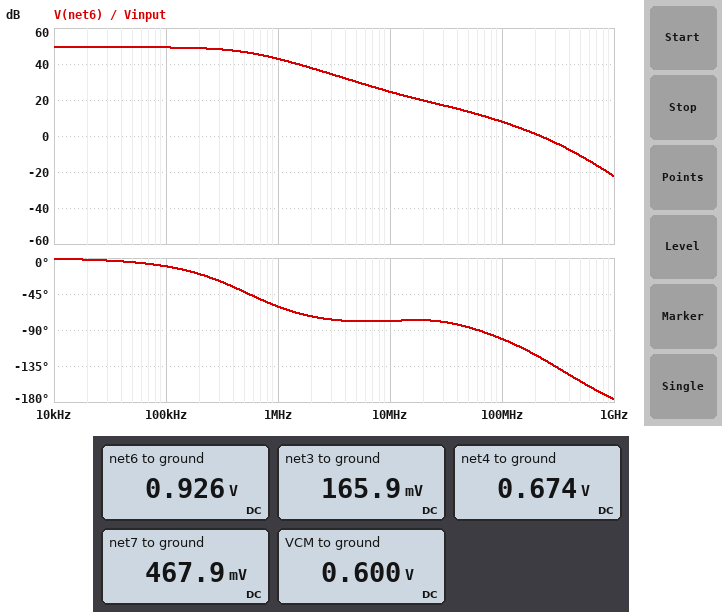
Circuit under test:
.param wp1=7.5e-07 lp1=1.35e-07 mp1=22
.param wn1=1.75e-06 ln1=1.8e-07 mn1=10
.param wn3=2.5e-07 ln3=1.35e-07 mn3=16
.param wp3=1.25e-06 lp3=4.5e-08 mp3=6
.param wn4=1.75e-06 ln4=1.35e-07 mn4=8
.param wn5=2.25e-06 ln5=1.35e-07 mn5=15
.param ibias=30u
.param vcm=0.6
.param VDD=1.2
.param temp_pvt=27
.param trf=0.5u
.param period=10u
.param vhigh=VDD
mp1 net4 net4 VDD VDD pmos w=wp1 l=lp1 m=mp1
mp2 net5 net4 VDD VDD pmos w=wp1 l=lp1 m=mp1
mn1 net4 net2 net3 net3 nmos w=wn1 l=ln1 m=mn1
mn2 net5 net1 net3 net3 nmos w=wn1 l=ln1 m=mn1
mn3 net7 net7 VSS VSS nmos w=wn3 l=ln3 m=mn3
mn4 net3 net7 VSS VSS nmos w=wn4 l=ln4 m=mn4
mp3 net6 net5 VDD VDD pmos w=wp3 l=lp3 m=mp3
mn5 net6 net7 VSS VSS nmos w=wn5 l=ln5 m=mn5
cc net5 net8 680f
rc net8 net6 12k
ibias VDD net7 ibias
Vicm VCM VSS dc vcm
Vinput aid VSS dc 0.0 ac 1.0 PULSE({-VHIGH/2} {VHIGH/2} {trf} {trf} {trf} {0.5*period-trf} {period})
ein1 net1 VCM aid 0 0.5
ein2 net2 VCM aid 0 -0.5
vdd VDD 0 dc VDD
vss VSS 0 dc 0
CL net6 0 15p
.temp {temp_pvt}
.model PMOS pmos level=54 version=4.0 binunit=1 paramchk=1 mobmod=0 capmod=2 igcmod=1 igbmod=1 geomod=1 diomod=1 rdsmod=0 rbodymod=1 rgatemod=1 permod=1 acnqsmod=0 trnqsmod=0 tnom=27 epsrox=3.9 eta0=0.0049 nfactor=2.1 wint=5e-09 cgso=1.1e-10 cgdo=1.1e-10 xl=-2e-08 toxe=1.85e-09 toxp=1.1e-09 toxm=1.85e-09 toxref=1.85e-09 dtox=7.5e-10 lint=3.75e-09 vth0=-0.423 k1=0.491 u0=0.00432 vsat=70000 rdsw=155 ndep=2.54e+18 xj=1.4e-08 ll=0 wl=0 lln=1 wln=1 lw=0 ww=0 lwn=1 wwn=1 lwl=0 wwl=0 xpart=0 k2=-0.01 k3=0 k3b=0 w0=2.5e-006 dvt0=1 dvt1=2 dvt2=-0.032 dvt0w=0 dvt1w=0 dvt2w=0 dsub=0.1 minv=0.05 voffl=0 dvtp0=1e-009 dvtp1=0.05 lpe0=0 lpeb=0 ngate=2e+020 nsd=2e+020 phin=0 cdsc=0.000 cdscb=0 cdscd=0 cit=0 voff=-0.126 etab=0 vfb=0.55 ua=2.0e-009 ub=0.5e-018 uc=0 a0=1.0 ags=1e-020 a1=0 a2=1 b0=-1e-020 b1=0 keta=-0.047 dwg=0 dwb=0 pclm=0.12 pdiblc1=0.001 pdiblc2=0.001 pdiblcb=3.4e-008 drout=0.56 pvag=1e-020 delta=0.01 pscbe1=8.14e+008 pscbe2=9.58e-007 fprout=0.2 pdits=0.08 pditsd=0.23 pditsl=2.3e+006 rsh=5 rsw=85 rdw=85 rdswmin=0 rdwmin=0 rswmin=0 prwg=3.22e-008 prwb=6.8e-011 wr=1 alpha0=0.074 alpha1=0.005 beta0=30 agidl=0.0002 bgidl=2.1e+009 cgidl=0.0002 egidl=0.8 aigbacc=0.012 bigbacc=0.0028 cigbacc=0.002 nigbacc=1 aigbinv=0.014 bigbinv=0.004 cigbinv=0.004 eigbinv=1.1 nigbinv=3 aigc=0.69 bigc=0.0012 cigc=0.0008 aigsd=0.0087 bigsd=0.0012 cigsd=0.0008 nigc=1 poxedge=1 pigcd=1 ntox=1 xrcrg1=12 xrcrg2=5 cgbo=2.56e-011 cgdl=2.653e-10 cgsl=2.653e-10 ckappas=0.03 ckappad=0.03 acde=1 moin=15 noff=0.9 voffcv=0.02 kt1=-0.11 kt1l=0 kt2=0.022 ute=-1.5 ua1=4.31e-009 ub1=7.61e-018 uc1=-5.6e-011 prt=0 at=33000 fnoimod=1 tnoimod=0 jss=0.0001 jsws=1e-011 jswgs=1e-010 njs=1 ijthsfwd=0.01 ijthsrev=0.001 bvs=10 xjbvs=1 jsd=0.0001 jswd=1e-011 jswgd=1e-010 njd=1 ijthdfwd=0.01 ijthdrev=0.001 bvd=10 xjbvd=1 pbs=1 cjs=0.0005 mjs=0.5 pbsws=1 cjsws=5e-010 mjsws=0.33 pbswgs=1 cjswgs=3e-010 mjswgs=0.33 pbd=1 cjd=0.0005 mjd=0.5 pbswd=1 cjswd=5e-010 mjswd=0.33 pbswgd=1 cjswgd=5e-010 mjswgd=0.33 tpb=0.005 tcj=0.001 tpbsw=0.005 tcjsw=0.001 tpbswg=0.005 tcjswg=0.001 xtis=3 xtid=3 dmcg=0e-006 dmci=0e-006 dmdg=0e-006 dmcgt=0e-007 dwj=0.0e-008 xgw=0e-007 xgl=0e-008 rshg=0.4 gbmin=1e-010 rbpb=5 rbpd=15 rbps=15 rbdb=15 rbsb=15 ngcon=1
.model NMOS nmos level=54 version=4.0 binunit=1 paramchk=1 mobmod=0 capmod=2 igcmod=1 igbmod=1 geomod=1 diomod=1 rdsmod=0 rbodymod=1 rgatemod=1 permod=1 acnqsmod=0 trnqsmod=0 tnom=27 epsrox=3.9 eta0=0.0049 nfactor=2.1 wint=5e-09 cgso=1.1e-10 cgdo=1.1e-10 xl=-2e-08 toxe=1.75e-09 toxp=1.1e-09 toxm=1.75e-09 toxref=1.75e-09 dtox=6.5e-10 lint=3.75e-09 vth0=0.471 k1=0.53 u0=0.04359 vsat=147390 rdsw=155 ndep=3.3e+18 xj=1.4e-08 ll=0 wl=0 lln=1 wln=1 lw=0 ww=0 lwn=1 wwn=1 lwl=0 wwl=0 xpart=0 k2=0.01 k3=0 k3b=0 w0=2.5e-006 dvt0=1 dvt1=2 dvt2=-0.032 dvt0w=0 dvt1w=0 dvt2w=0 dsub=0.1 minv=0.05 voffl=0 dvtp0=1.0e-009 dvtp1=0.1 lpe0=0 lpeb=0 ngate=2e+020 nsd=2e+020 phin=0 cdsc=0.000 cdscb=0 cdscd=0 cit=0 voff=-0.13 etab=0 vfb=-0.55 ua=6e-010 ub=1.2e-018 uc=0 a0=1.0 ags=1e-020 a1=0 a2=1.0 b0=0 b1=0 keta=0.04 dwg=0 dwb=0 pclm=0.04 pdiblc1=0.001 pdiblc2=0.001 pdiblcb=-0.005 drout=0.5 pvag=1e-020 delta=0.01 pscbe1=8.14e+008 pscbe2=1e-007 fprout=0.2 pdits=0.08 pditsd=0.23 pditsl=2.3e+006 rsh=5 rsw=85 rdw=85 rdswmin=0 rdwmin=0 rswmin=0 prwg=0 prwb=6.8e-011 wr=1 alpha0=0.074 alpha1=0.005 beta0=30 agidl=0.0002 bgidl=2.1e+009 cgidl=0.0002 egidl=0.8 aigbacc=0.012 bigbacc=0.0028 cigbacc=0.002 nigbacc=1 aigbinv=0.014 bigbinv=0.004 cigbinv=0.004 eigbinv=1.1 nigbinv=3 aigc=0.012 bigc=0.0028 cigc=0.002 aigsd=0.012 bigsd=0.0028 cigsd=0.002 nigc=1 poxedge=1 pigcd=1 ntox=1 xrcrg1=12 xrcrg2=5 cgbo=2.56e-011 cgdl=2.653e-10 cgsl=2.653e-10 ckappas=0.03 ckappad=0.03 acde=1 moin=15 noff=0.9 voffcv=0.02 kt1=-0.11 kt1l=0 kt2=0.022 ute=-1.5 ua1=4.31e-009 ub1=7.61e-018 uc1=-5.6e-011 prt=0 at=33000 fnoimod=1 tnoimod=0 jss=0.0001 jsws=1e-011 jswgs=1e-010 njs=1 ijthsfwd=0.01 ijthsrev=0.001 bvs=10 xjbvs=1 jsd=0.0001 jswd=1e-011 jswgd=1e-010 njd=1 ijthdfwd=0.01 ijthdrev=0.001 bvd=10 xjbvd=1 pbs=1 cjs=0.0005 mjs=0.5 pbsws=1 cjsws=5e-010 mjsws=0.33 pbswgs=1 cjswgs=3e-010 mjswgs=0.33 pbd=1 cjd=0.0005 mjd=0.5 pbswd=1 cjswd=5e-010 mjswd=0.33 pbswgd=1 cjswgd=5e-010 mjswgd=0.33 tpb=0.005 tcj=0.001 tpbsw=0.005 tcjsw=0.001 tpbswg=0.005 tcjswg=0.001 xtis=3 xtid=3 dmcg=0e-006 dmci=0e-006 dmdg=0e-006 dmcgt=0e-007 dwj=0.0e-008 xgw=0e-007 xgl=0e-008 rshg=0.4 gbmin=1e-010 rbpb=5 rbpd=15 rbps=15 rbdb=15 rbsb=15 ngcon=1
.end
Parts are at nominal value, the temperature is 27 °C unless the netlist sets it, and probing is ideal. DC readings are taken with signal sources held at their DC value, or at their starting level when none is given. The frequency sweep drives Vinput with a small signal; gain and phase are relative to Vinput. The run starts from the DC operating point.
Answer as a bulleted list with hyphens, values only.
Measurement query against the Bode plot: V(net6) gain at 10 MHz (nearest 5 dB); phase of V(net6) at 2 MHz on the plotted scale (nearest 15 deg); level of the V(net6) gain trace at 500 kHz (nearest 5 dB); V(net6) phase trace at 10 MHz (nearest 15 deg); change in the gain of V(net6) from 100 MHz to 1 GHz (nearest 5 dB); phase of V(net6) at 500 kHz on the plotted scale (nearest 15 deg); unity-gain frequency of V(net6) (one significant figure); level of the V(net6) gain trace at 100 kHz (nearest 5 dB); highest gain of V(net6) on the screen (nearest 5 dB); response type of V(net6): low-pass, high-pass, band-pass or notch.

- 25 dB
- -75 deg
- 45 dB
- -75 deg
- -30 dB
- -45 deg
- 200 MHz
- 50 dB
- 50 dB
- low-pass
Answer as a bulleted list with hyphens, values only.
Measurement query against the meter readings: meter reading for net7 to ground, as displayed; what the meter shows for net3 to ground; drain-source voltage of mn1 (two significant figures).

- 467.9 mV
- 165.9 mV
- 510 mV
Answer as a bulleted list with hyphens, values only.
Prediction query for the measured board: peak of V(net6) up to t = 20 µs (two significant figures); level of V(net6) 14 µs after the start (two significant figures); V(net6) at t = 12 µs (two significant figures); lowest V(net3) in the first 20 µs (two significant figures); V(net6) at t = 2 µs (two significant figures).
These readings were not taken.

- 1.2 V
- 1.2 V
- 1.2 V
- 3.1 mV
- 1.2 V
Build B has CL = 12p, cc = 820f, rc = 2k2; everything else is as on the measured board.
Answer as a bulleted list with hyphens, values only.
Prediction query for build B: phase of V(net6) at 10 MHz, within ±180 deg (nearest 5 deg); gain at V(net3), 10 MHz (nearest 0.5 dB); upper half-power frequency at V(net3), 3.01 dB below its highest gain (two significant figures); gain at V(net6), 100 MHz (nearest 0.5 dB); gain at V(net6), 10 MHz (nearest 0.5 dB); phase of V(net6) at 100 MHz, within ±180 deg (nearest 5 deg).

- -95 deg
- -32.0 dB
- 470 kHz
- -2.5 dB
- 22.5 dB
- -120 deg
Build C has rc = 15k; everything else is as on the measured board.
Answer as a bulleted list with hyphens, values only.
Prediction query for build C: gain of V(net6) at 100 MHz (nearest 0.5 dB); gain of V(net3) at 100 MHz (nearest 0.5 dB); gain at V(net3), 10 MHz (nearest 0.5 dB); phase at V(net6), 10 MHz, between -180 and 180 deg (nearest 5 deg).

- 9.5 dB
- -24.0 dB
- -28.5 dB
- -75 deg
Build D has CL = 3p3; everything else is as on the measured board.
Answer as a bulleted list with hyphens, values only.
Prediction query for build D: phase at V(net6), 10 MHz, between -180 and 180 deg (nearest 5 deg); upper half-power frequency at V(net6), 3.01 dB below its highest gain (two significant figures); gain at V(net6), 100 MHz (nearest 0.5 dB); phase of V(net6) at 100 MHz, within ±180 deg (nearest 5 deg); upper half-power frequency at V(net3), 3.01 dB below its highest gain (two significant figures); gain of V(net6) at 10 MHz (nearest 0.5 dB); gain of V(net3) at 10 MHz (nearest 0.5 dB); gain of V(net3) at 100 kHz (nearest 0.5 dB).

- -65 deg
- 560 kHz
- 17.0 dB
- -60 deg
- 570 kHz
- 25.5 dB
- -31.5 dB
- -13.5 dB
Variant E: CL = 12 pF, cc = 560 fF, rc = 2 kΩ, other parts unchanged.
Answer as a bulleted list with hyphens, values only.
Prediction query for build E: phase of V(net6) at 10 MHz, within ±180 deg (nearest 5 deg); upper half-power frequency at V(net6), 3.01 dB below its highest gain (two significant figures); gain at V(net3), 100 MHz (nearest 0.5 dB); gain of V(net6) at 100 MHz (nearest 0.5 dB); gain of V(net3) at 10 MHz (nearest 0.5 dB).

- -95 deg
- 670 kHz
- -35.5 dB
- -1.0 dB
- -28.5 dB
